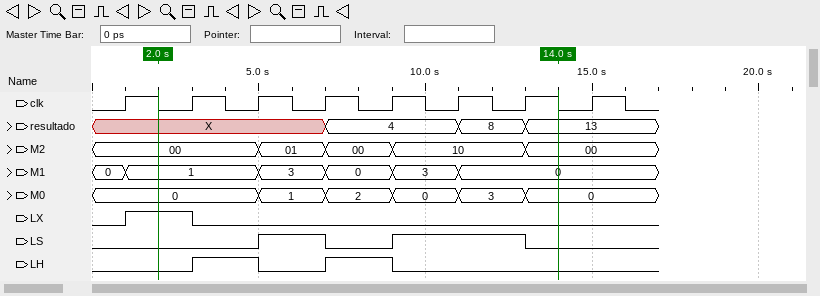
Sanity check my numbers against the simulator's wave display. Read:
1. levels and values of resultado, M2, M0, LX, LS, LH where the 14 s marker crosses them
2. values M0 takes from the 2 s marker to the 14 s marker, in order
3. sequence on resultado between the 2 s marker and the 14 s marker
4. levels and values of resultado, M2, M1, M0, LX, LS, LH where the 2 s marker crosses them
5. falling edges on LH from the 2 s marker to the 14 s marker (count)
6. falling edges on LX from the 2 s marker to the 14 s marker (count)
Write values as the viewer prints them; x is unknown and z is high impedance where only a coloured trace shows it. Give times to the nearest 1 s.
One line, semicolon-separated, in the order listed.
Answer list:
resultado=13, M2=00, M0=0, LX=0, LS=0, LH=0; 0, 1, 2, 0, 3, 0; X, 4, 8, 13; resultado=X, M2=00, M1=1, M0=0, LX=1, LS=0, LH=0; 2; 1
